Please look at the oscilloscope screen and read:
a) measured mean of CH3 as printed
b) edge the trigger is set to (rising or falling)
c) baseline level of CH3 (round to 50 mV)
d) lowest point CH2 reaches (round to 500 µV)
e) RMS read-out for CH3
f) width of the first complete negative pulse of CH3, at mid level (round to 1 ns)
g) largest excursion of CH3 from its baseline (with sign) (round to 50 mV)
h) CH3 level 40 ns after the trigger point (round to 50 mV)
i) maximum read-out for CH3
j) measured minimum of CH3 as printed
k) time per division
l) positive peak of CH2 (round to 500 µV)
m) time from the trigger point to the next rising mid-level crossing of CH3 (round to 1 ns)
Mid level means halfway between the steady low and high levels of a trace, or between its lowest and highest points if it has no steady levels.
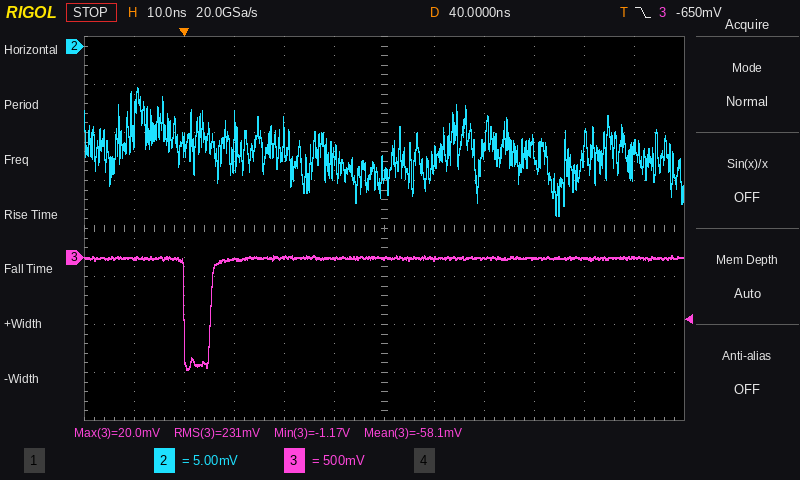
-58.1 mV
falling
0 mV
-17.5 mV
231 mV
5 ns
-1.15 V
0 mV
20.0 mV
-1.17 V
10 ns
-4.5 mV
5 ns
